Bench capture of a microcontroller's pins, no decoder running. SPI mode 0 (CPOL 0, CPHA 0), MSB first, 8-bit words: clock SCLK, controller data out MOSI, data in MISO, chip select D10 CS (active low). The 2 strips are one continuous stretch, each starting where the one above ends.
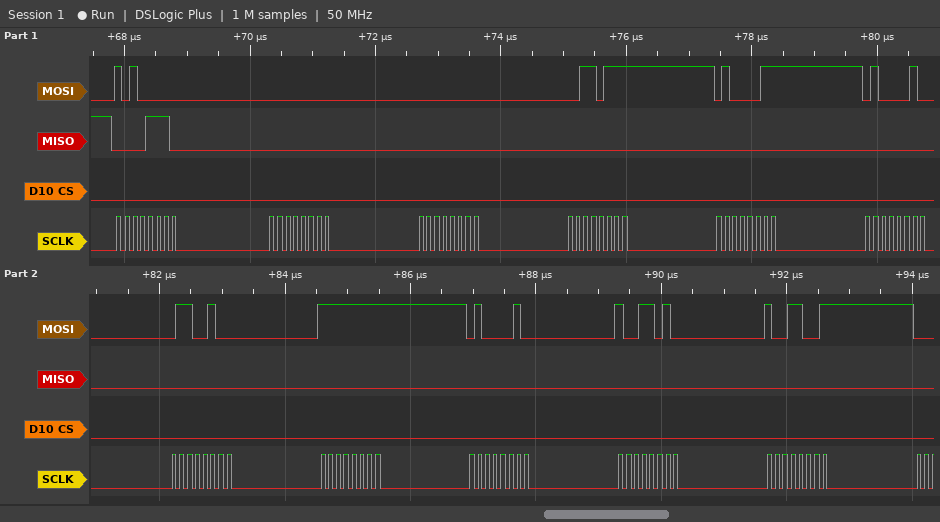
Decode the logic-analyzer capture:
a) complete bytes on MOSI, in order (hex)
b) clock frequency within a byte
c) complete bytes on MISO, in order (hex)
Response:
A0 00 00 37 43 42 64 FF 42 9A 99
8 MHz
0E 00 00 00 00 00 00 00 00 00 00
